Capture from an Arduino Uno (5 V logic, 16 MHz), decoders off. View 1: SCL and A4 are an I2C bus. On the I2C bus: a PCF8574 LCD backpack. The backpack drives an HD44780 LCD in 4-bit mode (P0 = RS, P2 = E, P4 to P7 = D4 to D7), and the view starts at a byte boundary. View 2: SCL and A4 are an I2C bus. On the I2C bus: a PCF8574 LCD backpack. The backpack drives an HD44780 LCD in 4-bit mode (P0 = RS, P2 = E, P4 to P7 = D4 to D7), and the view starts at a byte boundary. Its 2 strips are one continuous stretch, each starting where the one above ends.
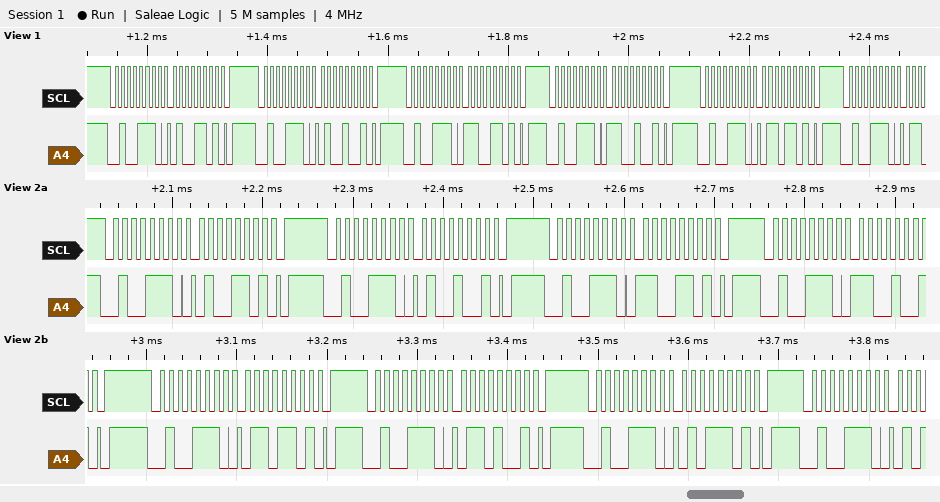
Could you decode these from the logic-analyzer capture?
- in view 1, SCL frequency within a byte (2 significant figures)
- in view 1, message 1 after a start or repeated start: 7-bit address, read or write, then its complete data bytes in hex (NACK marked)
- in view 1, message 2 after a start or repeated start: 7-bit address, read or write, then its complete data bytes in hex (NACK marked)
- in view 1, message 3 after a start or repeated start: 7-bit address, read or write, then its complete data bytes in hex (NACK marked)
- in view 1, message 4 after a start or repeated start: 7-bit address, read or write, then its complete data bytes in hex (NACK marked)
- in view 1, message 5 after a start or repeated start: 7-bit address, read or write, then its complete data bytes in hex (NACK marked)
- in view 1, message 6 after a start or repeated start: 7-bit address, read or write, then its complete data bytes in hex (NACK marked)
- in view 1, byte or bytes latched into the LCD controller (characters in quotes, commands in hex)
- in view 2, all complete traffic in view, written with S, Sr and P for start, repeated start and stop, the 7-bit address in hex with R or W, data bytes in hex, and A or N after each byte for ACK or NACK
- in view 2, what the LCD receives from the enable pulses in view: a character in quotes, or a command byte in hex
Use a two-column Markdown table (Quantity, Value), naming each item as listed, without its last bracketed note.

| Quantity | Value |
|---|---|
| in view 1, SCL frequency within a byte | 100 kHz |
| in view 1, message 1 after a start or repeated start: 7-bit address, read or write, then its complete data bytes in hex | 0x27 write: 4D |
| in view 1, message 2 after a start or repeated start: 7-bit address, read or write, then its complete data bytes in hex | 0x27 write: 49 |
| in view 1, message 3 after a start or repeated start: 7-bit address, read or write, then its complete data bytes in hex | 0x27 write: CD |
| in view 1, message 4 after a start or repeated start: 7-bit address, read or write, then its complete data bytes in hex | 0x27 write: C9 |
| in view 1, message 5 after a start or repeated start: 7-bit address, read or write, then its complete data bytes in hex | 0x27 write: 6D |
| in view 1, message 6 after a start or repeated start: 7-bit address, read or write, then its complete data bytes in hex | 0x27 write |
| in view 1, byte or bytes latched into the LCD controller | 'L' |
| in view 2, all complete traffic in view, written with S, Sr and P for start, repeated start and stop, the 7-bit address in hex with R or W, data bytes in hex, and A or N after each byte for ACK or NACK | S 27W A 4D A P S 27W A 49 A P S 27W A CD A P S 27W A C9 A P S 27W A 6D A P S 27W A 69 A P S 27W A 5D A P S 27W A |
| in view 2, what the LCD receives from the enable pulses in view: a character in quotes, or a command byte in hex | 'L' |
